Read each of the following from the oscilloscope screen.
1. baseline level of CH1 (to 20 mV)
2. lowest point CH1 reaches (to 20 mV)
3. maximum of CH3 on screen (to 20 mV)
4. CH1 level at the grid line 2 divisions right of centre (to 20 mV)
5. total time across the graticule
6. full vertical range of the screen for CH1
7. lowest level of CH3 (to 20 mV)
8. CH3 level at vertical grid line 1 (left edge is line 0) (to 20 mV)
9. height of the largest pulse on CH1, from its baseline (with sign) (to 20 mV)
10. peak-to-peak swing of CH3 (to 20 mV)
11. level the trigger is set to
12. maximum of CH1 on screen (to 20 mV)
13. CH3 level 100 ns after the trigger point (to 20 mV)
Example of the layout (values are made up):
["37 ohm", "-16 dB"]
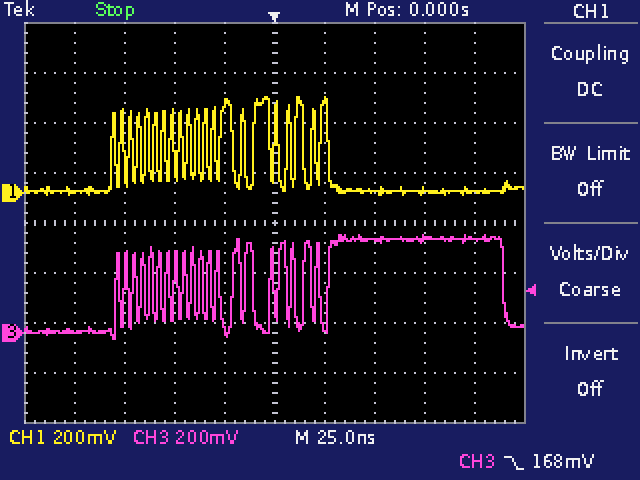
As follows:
["0 mV", "0 mV", "400 mV", "0 mV", "250 ns", "1.6 V", "-20 mV", "0 mV", "+380 mV", "420 mV", "168 mV", "380 mV", "380 mV"]
